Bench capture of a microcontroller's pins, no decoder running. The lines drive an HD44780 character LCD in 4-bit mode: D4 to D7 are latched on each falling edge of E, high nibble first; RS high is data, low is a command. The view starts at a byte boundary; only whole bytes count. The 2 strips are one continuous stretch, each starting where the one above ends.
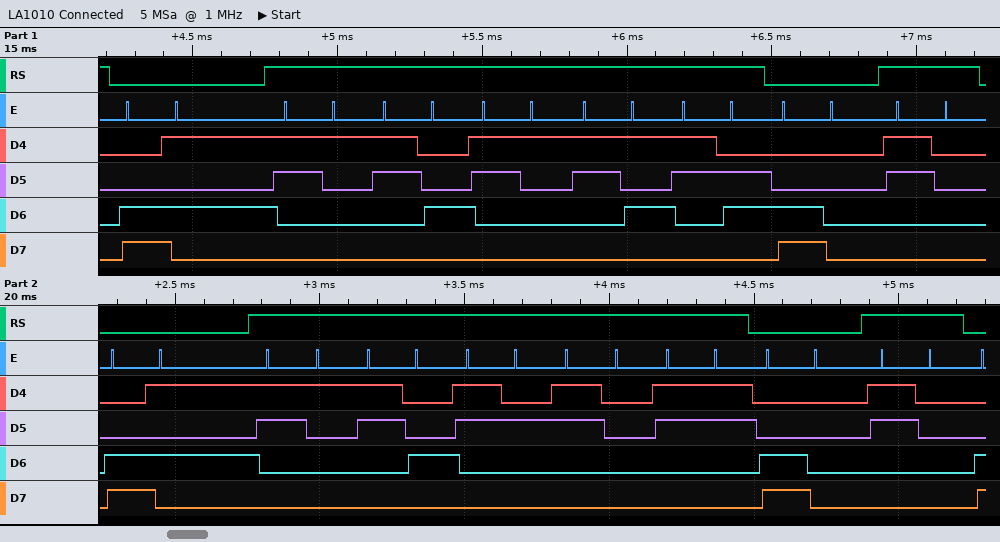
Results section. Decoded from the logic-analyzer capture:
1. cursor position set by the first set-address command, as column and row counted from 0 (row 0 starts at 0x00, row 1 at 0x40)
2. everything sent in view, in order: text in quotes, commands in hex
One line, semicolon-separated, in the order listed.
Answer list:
column 5, row 1; 0xC5 "14156" 0xC0 "0" 0xC5 "14203" 0xC0 "0"
